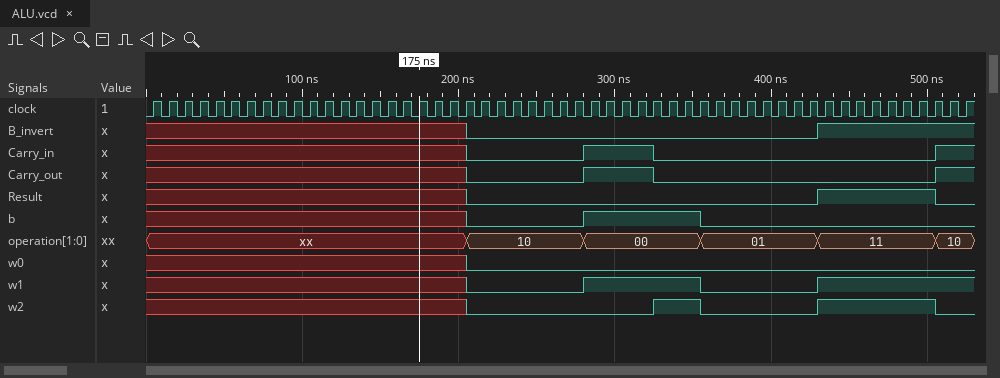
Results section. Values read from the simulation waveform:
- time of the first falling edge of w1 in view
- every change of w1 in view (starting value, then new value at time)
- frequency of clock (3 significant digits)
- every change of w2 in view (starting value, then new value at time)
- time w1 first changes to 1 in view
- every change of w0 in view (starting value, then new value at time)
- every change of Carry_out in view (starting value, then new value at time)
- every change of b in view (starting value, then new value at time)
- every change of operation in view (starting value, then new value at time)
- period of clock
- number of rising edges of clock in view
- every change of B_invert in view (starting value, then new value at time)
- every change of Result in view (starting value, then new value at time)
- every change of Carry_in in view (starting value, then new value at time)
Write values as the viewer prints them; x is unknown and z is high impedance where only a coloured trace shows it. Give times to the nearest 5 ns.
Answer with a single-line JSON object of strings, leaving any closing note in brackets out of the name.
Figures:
{"time of the first falling edge of w1 in view": "355 ns", "every change of w1 in view": "x, 0 at 205 ns, 1 at 280 ns, 0 at 355 ns, 1 at 430 ns", "frequency of clock": "100 MHz", "every change of w2 in view": "x, 0 at 205 ns, 1 at 325 ns, 0 at 355 ns, 1 at 430 ns, 0 at 505 ns", "time w1 first changes to 1 in view": "280 ns", "every change of w0 in view": "x, 0 at 205 ns", "every change of Carry_out in view": "x, 0 at 205 ns, 1 at 280 ns, 0 at 325 ns, 1 at 505 ns", "every change of b in view": "x, 0 at 205 ns, 1 at 280 ns, 0 at 355 ns", "every change of operation in view": "xx, 10 at 205 ns, 00 at 280 ns, 01 at 355 ns, 11 at 430 ns, 10 at 505 ns", "period of clock": "10 ns", "number of rising edges of clock in view": "53", "every change of B_invert in view": "x, 0 at 205 ns, 1 at 430 ns", "every change of Result in view": "x, 0 at 205 ns, 1 at 430 ns, 0 at 505 ns", "every change of Carry_in in view": "x, 0 at 205 ns, 1 at 280 ns, 0 at 325 ns, 1 at 505 ns"}
